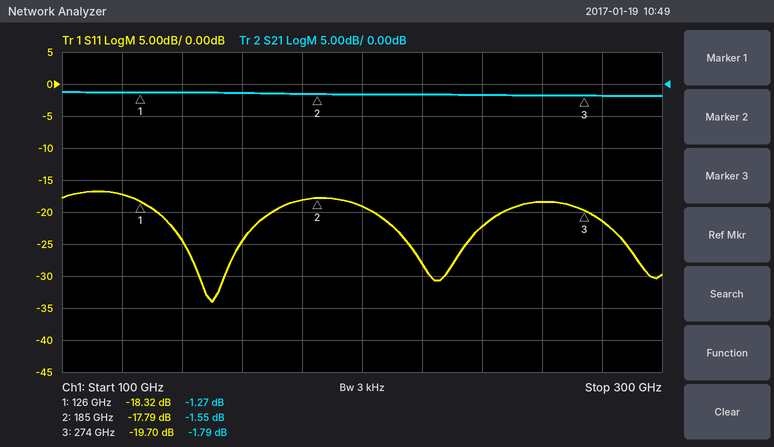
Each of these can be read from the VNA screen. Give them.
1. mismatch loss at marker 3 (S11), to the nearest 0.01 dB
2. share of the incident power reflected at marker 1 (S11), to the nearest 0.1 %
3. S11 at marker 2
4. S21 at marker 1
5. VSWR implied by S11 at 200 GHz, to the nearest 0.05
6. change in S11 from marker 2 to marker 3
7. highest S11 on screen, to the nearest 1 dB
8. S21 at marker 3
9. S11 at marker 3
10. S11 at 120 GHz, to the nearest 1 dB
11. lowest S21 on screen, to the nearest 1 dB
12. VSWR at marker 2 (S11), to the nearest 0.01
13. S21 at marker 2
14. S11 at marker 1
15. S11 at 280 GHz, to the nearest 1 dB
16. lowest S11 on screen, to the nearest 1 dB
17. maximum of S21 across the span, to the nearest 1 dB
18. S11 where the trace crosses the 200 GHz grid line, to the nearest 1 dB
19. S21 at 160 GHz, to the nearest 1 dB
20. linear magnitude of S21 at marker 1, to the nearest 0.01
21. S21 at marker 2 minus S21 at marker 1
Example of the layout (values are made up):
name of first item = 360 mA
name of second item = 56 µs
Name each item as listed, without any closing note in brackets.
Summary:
mismatch loss at marker 3 (S11), to the nearest 0.01 dB = 0.05 dB
share of the incident power reflected at marker 1 (S11), to the nearest 0.1 % = 1.5 %
S11 at marker 2 = -17.79 dB
S21 at marker 1 = -1.27 dB
VSWR implied by S11 at 200 GHz, to the nearest 0.05 = 1.25
change in S11 from marker 2 to marker 3 = -1.91 dB
highest S11 on screen, to the nearest 1 dB = -17 dB
S21 at marker 3 = -1.79 dB
S11 at marker 3 = -19.70 dB
S11 at 120 GHz, to the nearest 1 dB = -17 dB
lowest S21 on screen, to the nearest 1 dB = -2 dB
VSWR at marker 2 (S11), to the nearest 0.01 = 1.30
S21 at marker 2 = -1.55 dB
S11 at marker 1 = -18.32 dB
S11 at 280 GHz, to the nearest 1 dB = -21 dB
lowest S11 on screen, to the nearest 1 dB = -34 dB
maximum of S21 across the span, to the nearest 1 dB = -1 dB
S11 where the trace crosses the 200 GHz grid line, to the nearest 1 dB = -19 dB
S21 at 160 GHz, to the nearest 1 dB = -1 dB
linear magnitude of S21 at marker 1, to the nearest 0.01 = 0.86
S21 at marker 2 minus S21 at marker 1 = -0.28 dB
